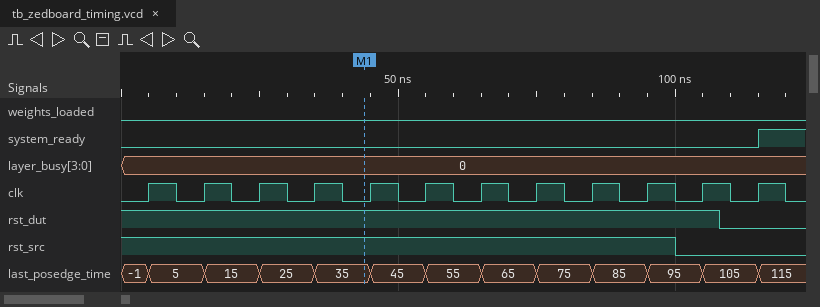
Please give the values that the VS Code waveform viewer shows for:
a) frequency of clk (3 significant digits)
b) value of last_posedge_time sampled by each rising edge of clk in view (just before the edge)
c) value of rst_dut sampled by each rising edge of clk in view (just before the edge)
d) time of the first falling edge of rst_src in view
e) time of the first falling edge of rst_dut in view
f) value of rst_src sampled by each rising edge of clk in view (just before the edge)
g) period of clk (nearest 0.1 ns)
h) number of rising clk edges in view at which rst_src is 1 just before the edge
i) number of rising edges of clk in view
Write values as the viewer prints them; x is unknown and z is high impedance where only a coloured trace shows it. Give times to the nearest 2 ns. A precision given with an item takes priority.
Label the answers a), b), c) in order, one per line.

a) 100 MHz
b) -1, 5, 15, 25, 35, 45, 55, 65, 75, 85, 95, 105
c) 1 1 1 1 1 1 1 1 1 1 1 0
d) 100 ns
e) 108 ns
f) 1 1 1 1 1 1 1 1 1 1 0 0
g) 10 ns
h) 10
i) 12
